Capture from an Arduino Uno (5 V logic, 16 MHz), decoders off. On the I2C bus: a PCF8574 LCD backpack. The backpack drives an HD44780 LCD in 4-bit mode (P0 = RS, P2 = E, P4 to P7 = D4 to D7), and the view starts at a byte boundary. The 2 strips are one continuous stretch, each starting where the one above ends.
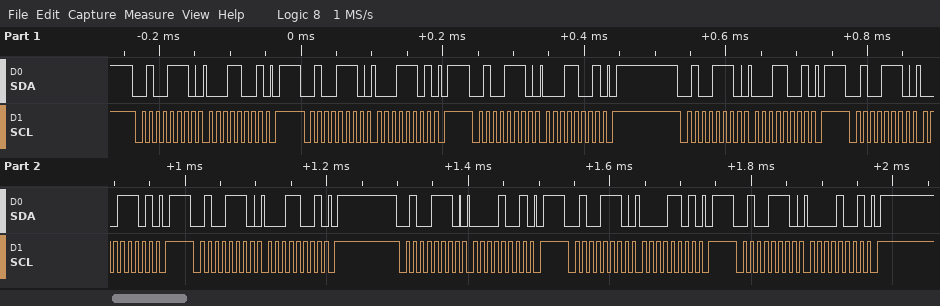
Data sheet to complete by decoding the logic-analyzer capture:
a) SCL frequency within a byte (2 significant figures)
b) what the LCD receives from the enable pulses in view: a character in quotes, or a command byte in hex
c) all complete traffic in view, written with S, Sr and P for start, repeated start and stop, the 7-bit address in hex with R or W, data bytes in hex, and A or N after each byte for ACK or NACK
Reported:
100 kHz
data 0x11
S 27W A 19 A P S 27W A 1D A P S 27W A 19 A P S 27W A 19 A P S 27W A 1D A P S 27W A 19 A P S 27W A 09 A P S 27W A 0D A P S 27W A 09 A P
